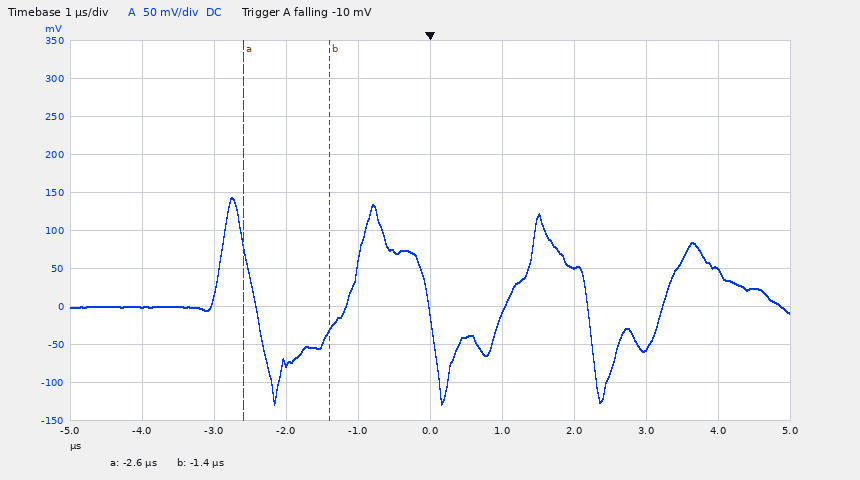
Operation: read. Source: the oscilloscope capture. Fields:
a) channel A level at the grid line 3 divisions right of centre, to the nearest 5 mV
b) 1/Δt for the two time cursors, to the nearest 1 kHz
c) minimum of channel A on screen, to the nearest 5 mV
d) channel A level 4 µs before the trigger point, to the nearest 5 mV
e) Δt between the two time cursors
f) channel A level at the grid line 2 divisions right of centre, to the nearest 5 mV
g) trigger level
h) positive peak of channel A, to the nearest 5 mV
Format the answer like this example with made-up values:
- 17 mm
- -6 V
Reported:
- -55 mV
- 833 kHz
- -130 mV
- 0 mV
- 1.2 µs
- 50 mV
- -10 mV
- 145 mV
